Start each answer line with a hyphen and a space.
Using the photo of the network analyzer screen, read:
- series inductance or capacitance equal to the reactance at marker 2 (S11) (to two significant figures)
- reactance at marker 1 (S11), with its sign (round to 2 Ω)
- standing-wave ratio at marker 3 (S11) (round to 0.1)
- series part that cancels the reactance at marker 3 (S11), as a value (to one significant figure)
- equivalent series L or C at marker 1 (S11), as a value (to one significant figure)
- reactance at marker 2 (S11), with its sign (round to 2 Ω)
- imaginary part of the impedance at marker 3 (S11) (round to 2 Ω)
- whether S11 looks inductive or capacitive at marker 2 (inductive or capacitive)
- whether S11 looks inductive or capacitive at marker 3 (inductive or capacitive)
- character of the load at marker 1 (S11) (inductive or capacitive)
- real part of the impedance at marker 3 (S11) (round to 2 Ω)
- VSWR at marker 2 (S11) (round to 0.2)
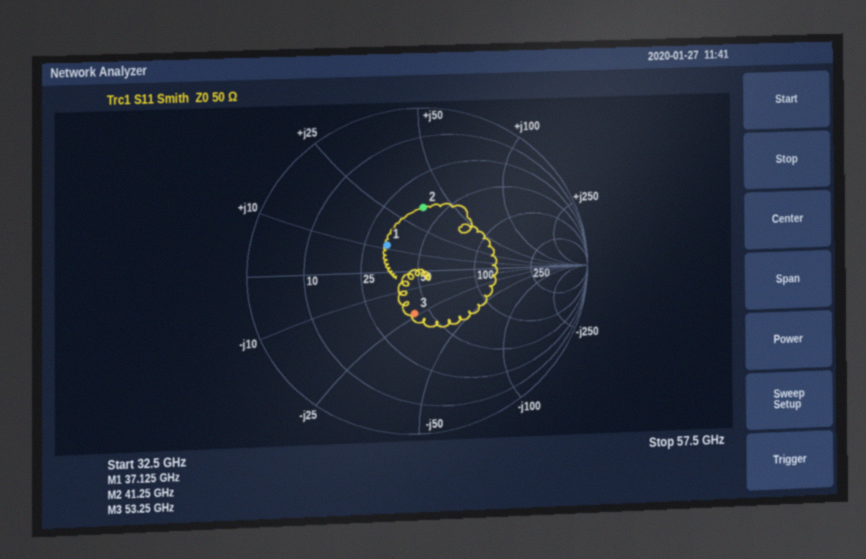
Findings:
- 140 pH
- +12 Ω
- 1.7
- 70 pH
- 50 pH
- +36 Ω
- -24 Ω
- inductive
- capacitive
- inductive
- 42 Ω
- 2.2
